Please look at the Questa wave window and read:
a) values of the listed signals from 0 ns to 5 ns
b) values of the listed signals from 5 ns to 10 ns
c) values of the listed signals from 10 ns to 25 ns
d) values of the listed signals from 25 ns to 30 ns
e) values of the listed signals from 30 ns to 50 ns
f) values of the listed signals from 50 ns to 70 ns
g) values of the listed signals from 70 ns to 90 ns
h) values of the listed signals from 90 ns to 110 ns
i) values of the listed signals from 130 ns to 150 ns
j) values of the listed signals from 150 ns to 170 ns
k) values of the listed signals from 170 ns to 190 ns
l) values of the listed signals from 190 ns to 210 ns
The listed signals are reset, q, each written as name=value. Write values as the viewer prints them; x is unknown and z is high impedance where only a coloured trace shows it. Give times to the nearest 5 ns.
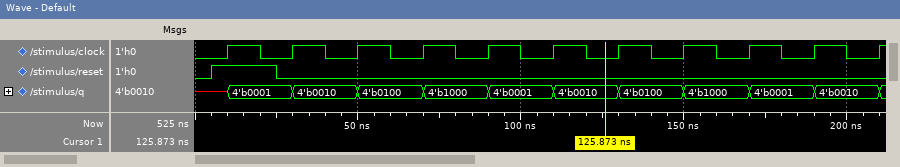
reset=0, q=x
reset=1, q=x
reset=1, q=4'b0001
reset=0, q=4'b0001
reset=0, q=4'b0010
reset=0, q=4'b0100
reset=0, q=4'b1000
reset=0, q=4'b0001
reset=0, q=4'b0100
reset=0, q=4'b1000
reset=0, q=4'b0001
reset=0, q=4'b0010
